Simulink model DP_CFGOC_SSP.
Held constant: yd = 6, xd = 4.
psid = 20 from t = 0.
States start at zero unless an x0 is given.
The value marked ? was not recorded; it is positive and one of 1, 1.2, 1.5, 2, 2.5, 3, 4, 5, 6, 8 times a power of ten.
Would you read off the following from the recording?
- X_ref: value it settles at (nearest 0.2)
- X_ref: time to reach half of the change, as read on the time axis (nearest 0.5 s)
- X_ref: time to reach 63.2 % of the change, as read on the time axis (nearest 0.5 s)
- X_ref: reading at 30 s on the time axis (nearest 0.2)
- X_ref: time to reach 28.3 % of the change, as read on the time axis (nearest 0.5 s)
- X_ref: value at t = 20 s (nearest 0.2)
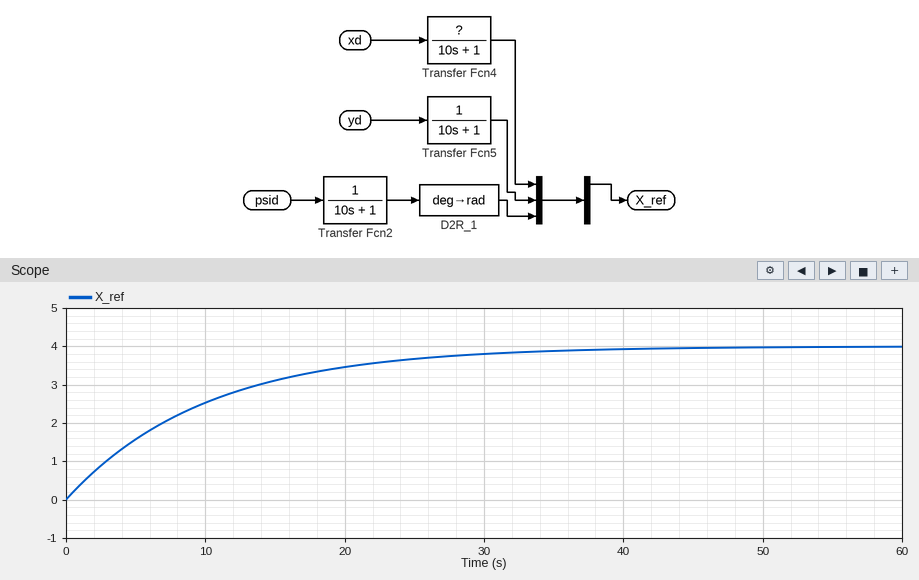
4.0
7.0 s
10.0 s
3.8
3.5 s
3.4
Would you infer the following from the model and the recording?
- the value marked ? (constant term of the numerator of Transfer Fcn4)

1
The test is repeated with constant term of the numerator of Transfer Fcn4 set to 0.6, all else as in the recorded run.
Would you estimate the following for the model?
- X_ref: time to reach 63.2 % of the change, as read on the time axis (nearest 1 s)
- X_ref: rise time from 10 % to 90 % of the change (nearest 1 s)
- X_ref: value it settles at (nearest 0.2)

10 s
22 s
2.4
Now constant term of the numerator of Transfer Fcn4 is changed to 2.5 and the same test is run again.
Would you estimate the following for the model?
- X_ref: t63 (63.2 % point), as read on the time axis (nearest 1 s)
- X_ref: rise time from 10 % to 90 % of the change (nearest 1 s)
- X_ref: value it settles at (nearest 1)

10 s
22 s
10
